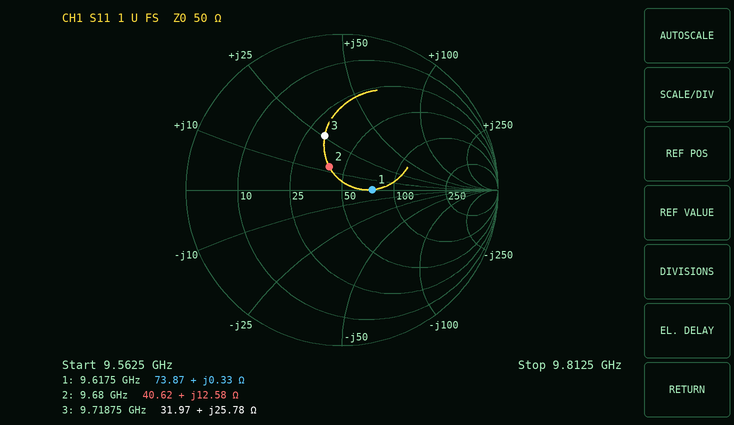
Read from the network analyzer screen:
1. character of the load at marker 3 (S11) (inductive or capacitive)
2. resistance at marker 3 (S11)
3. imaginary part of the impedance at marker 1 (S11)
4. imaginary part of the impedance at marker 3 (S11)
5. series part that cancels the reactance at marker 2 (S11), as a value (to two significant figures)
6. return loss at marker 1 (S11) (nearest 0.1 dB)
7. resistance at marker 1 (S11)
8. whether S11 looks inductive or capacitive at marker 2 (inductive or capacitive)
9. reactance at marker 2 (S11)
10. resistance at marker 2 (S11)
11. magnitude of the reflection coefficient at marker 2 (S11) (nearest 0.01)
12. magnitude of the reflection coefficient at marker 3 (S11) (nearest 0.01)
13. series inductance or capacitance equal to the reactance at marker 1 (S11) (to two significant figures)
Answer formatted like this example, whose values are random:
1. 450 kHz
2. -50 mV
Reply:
1. inductive
2. 31.97 Ω
3. +0.33 Ω
4. +25.78 Ω
5. 1.3 pF
6. 14.3 dB
7. 73.87 Ω
8. inductive
9. +12.58 Ω
10. 40.62 Ω
11. 0.17
12. 0.37
13. 5.5 pH
